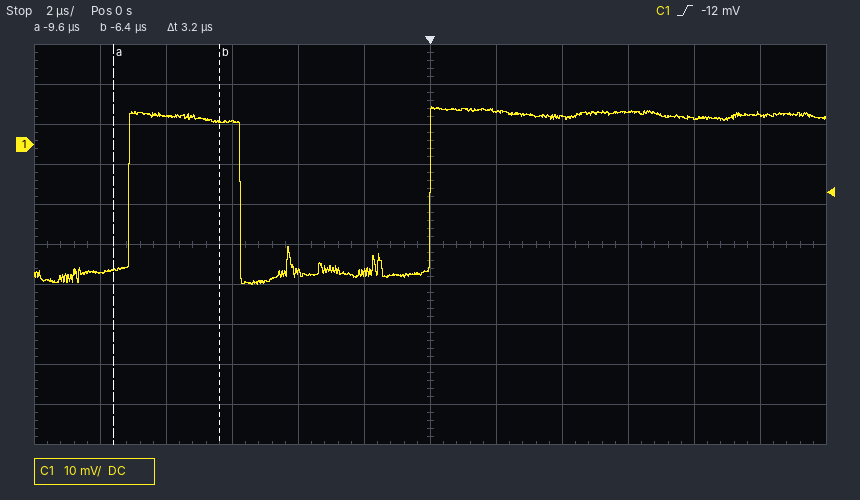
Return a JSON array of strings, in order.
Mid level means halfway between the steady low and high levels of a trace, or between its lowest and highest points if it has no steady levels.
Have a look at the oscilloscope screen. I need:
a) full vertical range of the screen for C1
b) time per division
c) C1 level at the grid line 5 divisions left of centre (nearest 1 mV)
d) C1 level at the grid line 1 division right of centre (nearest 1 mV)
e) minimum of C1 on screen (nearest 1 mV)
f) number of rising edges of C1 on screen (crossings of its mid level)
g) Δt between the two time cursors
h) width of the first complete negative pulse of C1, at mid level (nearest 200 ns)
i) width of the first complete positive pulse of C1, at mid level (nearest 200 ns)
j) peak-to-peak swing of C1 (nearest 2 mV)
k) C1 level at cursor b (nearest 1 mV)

["100 mV", "2 µs", "-32 mV", "8 mV", "-35 mV", "2", "3.2 µs", "5.8 µs", "3.4 µs", "44 mV", "6 mV"]
